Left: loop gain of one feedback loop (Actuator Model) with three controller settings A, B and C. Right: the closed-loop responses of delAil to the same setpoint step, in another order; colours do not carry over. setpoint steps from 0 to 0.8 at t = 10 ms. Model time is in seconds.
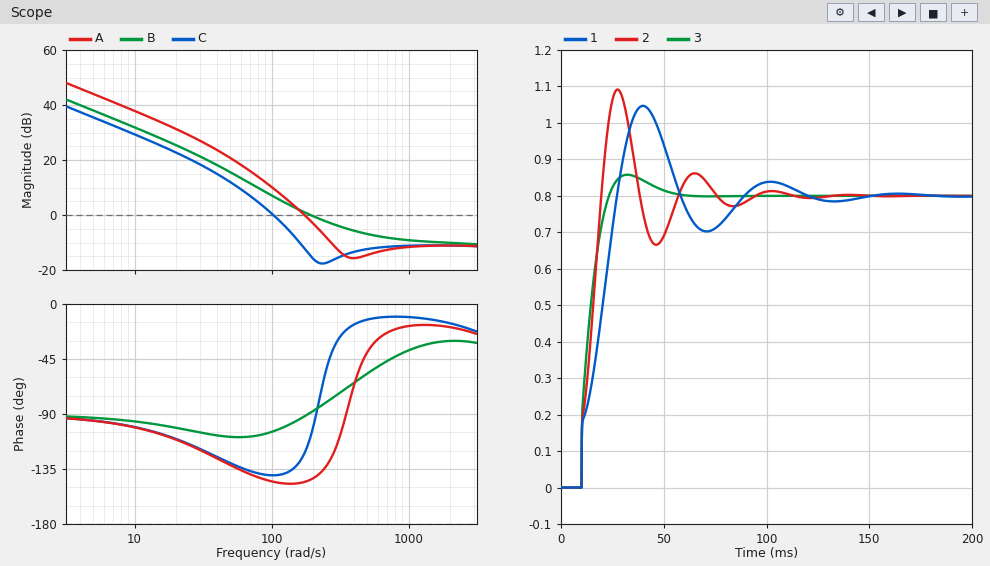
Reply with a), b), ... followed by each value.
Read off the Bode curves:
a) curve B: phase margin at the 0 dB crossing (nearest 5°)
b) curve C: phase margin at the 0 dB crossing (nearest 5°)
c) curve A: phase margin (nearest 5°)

a) 90°
b) 40°
c) 35°
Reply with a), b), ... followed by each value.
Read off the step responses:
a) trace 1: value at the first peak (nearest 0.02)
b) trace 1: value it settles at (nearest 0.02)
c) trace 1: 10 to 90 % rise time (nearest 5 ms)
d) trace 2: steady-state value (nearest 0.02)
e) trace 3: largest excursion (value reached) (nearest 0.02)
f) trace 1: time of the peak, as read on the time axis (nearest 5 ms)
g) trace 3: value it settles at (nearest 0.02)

a) 1.04
b) 0.80
c) 15 ms
d) 0.80
e) 0.86
f) 40 ms
g) 0.80
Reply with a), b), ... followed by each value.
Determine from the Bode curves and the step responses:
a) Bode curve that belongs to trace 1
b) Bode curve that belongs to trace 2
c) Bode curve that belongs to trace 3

a) C
b) A
c) B
